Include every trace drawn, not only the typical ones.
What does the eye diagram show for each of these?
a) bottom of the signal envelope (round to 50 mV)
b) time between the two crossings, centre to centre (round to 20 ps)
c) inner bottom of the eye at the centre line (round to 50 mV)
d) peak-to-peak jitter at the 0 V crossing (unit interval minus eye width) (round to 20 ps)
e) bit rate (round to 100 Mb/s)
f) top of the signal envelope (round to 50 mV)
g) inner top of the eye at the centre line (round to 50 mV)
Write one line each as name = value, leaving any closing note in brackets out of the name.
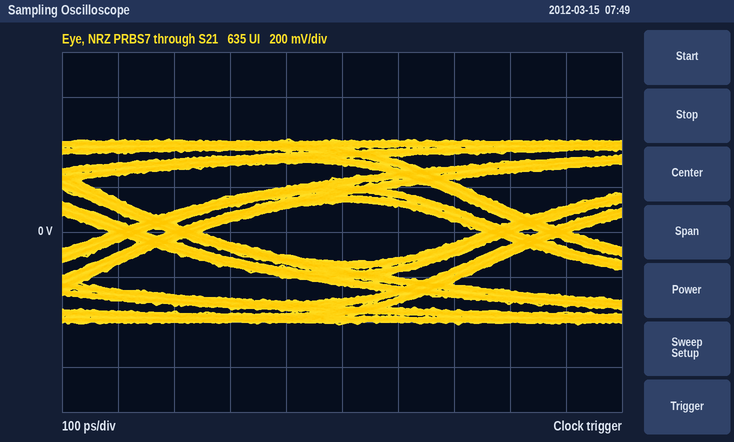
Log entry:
bottom of the signal envelope = -400 mV
time between the two crossings, centre to centre = 660 ps
inner bottom of the eye at the centre line = -150 mV
peak-to-peak jitter at the 0 V crossing (unit interval minus eye width) = 160 ps
bit rate = 1.5 Gb/s
top of the signal envelope = 400 mV
inner top of the eye at the centre line = 150 mV
